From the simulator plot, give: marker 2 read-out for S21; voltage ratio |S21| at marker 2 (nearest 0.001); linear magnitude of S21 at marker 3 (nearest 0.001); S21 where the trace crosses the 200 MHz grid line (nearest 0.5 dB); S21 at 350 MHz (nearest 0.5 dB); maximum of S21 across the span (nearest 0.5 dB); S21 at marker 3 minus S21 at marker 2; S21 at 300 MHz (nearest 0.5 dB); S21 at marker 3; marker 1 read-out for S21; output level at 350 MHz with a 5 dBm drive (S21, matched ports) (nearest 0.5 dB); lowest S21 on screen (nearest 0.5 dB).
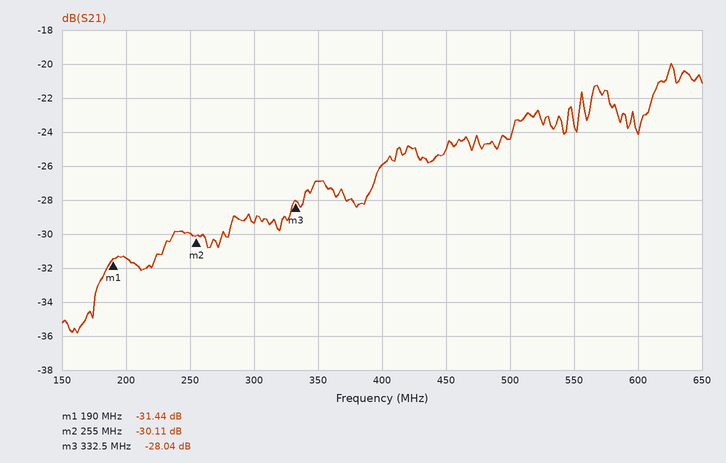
-30.11 dB
0.031
0.040
-31.5 dB
-27.0 dB
-20.0 dB
2.07 dB
-29.5 dB
-28.04 dB
-31.44 dB
-22.0 dBm
-36.0 dB
